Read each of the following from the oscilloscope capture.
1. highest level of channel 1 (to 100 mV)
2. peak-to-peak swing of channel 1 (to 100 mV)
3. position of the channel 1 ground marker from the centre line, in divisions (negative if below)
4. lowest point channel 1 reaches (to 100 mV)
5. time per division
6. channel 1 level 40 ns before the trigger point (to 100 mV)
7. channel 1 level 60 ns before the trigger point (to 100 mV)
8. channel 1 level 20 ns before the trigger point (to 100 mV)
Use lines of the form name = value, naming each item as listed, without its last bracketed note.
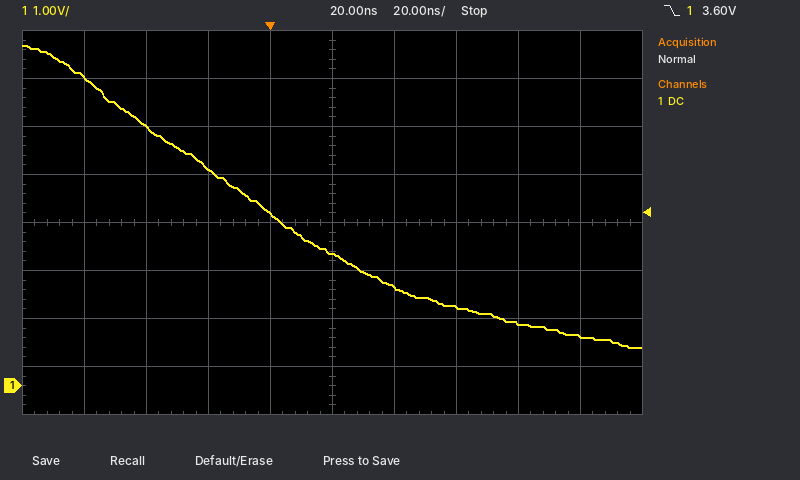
highest level of channel 1 = 7.1 V
peak-to-peak swing of channel 1 = 6.3 V
position of the channel 1 ground marker from the centre line, in divisions = -3.4 div
lowest point channel 1 reaches = 800 mV
time per division = 20 ns
channel 1 level 40 ns before the trigger point = 5.4 V
channel 1 level 60 ns before the trigger point = 6.4 V
channel 1 level 20 ns before the trigger point = 4.5 V
